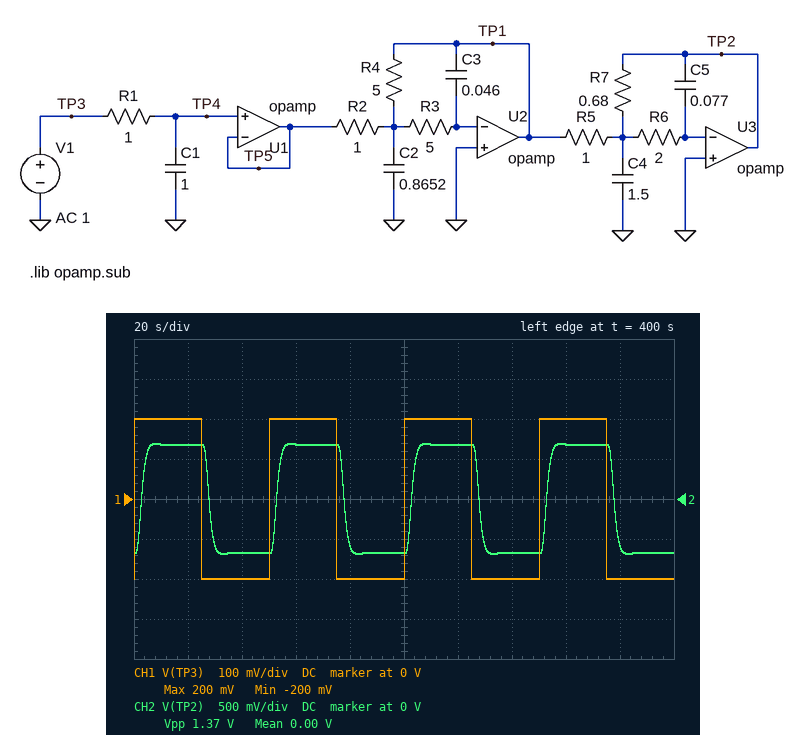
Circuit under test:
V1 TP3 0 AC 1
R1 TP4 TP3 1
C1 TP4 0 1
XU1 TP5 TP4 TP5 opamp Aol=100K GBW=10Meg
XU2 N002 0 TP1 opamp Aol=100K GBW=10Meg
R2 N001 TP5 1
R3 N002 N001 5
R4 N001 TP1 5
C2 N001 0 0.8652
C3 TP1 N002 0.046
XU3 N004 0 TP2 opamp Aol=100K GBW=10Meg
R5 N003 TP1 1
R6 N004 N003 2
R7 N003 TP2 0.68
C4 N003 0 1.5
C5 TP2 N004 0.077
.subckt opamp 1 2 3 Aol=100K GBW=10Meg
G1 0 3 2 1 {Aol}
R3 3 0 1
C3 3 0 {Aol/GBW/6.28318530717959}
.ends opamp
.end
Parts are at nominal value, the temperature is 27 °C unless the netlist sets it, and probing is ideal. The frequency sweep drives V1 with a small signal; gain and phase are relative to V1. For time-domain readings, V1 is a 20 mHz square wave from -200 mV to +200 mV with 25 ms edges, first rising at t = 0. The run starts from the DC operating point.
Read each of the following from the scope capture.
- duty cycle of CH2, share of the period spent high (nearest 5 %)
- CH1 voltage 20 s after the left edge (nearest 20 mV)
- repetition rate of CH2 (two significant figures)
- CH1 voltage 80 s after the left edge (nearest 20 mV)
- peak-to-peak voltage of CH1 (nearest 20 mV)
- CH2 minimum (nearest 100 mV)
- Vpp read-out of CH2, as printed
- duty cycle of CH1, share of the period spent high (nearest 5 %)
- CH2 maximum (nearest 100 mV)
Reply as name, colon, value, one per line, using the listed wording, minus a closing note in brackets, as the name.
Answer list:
duty cycle of CH2, share of the period spent high: 50 %
CH1 voltage 20 s after the left edge: 200 mV
repetition rate of CH2: 20 mHz
CH1 voltage 80 s after the left edge: -200 mV
peak-to-peak voltage of CH1: 400 mV
CH2 minimum: -700 mV
Vpp read-out of CH2, as printed: 1.37 V
duty cycle of CH1, share of the period spent high: 50 %
CH2 maximum: 700 mV
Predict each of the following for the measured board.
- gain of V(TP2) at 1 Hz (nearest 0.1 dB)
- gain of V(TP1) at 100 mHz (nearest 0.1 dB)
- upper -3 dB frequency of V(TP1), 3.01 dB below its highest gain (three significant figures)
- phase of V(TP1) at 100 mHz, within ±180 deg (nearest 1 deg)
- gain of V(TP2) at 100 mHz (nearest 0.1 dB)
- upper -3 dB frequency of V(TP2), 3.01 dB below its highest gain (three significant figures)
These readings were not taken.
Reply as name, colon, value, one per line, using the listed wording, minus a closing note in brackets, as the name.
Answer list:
gain of V(TP2) at 1 Hz: -52.3 dB
gain of V(TP1) at 100 mHz: 11.1 dB
upper -3 dB frequency of V(TP1), 3.01 dB below its highest gain: 102 mHz
phase of V(TP1) at 100 mHz, within ±180 deg: 89 deg
gain of V(TP2) at 100 mHz: 8.1 dB
upper -3 dB frequency of V(TP2), 3.01 dB below its highest gain: 109 mHz
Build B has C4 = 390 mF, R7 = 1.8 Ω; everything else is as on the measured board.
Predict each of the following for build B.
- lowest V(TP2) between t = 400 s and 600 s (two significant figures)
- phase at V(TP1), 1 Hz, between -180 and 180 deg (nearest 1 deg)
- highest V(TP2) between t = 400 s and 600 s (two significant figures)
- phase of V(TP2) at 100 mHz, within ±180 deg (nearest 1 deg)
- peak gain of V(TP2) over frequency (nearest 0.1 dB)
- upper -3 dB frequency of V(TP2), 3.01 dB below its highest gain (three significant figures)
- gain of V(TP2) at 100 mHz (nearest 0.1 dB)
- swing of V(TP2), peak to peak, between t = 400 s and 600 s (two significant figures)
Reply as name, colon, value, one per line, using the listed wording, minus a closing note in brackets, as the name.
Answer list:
lowest V(TP2) between t = 400 s and 600 s: -1.8 V
phase at V(TP1), 1 Hz, between -180 and 180 deg: -66 deg
highest V(TP2) between t = 400 s and 600 s: 1.8 V
phase of V(TP2) at 100 mHz, within ±180 deg: -112 deg
peak gain of V(TP2) over frequency: 19.1 dB
upper -3 dB frequency of V(TP2), 3.01 dB below its highest gain: 99.0 mHz
gain of V(TP2) at 100 mHz: 16.0 dB
swing of V(TP2), peak to peak, between t = 400 s and 600 s: 3.6 V
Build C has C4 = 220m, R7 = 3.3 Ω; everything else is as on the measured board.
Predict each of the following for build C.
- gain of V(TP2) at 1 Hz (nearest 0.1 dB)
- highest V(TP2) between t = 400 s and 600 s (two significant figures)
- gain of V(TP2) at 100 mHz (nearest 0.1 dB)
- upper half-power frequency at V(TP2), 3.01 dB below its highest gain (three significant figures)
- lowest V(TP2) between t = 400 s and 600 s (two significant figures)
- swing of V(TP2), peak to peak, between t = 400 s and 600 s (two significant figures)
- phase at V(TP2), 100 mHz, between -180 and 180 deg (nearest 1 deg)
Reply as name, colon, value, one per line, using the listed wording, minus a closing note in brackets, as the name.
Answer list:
gain of V(TP2) at 1 Hz: -40.2 dB
highest V(TP2) between t = 400 s and 600 s: 3.3 V
gain of V(TP2) at 100 mHz: 20.5 dB
upper half-power frequency at V(TP2), 3.01 dB below its highest gain: 88.6 mHz
lowest V(TP2) between t = 400 s and 600 s: -3.3 V
swing of V(TP2), peak to peak, between t = 400 s and 600 s: 6.6 V
phase at V(TP2), 100 mHz, between -180 and 180 deg: -122 deg
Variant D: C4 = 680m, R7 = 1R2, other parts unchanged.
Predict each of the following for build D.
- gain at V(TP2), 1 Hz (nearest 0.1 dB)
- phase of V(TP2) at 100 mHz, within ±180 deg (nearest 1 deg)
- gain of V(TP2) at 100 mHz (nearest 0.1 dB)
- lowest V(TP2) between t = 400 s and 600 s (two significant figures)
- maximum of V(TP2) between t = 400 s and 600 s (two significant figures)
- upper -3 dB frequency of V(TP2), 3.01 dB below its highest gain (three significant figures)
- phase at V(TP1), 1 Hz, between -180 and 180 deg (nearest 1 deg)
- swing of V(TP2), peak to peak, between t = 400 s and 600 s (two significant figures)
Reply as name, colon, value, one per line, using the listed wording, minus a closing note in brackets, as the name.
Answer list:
gain at V(TP2), 1 Hz: -46.1 dB
phase of V(TP2) at 100 mHz, within ±180 deg: -107 deg
gain of V(TP2) at 100 mHz: 12.8 dB
lowest V(TP2) between t = 400 s and 600 s: -1.2 V
maximum of V(TP2) between t = 400 s and 600 s: 1.2 V
upper -3 dB frequency of V(TP2), 3.01 dB below its highest gain: 104 mHz
phase at V(TP1), 1 Hz, between -180 and 180 deg: -66 deg
swing of V(TP2), peak to peak, between t = 400 s and 600 s: 2.4 V
